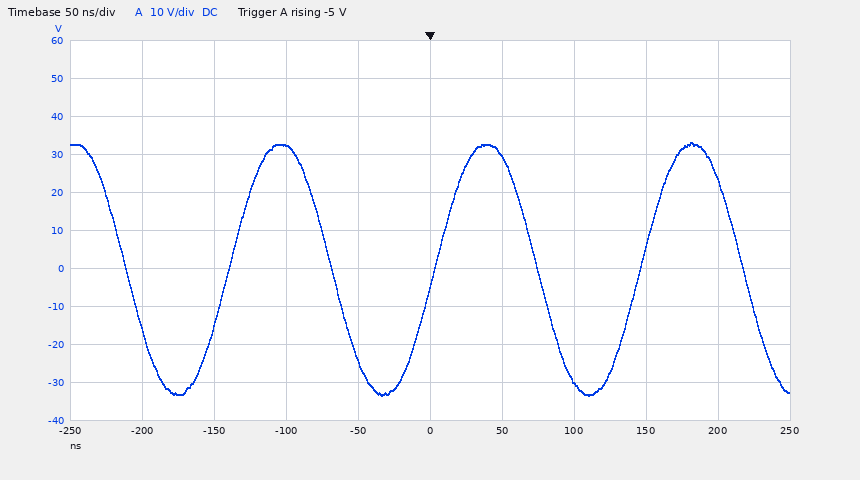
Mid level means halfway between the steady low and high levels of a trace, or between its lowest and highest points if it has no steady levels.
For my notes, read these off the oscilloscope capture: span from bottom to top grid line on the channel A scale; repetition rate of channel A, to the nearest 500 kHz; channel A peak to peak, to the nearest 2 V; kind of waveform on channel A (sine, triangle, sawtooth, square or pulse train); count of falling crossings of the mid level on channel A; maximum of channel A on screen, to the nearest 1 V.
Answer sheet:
100 V
7.0 MHz
66 V
sine
4
33 V
